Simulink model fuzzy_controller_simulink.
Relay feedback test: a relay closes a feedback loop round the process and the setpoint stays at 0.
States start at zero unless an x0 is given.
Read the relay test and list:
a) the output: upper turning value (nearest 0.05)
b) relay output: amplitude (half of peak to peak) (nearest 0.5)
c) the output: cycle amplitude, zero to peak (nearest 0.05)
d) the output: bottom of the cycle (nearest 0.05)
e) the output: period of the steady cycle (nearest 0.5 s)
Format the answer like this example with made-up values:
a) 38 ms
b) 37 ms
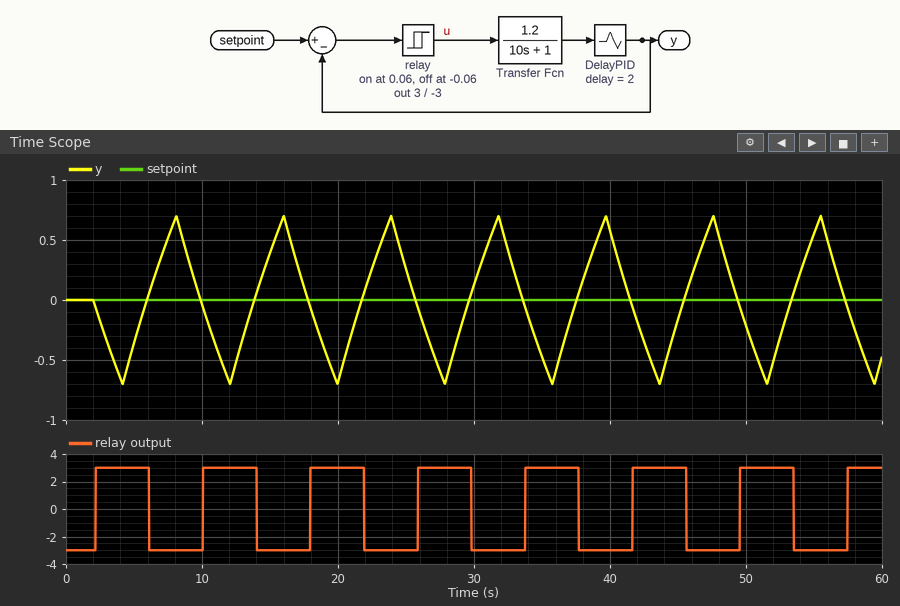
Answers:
a) 0.70
b) 3.0
c) 0.70
d) -0.70
e) 8.0 s
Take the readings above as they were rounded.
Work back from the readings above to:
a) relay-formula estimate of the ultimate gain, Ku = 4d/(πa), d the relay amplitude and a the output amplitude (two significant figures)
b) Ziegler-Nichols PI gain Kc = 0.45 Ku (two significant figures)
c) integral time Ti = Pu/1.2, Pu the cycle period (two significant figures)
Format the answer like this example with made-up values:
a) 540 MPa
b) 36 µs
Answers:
a) 5.5
b) 2.5
c) 6.7 s
